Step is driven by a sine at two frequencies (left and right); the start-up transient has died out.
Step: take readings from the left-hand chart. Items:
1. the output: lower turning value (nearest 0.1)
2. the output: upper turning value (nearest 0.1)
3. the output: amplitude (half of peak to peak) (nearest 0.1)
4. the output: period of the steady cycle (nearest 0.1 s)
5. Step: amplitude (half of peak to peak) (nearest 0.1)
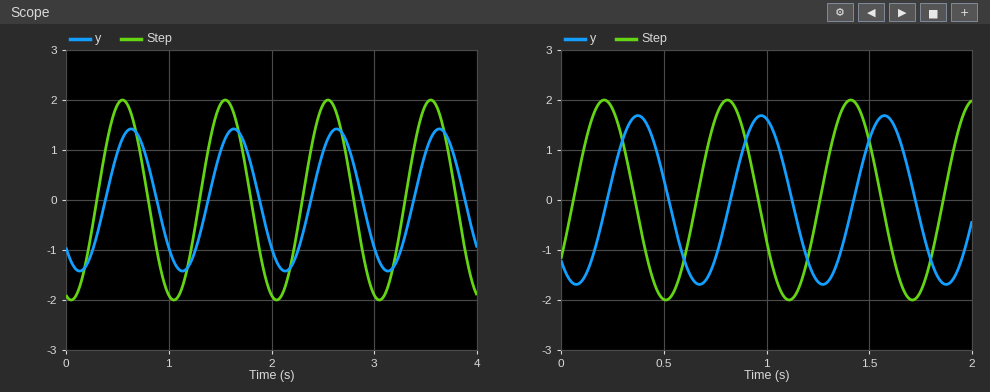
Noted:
-1.4
1.4
1.4
1.0 s
2.0
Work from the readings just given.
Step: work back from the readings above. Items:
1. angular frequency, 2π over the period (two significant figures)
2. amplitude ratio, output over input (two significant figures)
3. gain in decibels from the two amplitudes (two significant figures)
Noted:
6.3 rad/s
0.70
-3.1 dB
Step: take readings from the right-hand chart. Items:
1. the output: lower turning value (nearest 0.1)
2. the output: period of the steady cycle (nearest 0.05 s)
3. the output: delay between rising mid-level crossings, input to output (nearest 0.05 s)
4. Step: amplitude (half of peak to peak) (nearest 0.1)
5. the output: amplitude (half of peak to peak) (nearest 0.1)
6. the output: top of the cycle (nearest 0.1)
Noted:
-1.7
0.60 s
0.15 s
2.0
1.7
1.7
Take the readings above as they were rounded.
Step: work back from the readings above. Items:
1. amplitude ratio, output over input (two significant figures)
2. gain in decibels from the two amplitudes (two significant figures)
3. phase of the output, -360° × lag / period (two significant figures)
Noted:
0.85
-1.4 dB
-90°
